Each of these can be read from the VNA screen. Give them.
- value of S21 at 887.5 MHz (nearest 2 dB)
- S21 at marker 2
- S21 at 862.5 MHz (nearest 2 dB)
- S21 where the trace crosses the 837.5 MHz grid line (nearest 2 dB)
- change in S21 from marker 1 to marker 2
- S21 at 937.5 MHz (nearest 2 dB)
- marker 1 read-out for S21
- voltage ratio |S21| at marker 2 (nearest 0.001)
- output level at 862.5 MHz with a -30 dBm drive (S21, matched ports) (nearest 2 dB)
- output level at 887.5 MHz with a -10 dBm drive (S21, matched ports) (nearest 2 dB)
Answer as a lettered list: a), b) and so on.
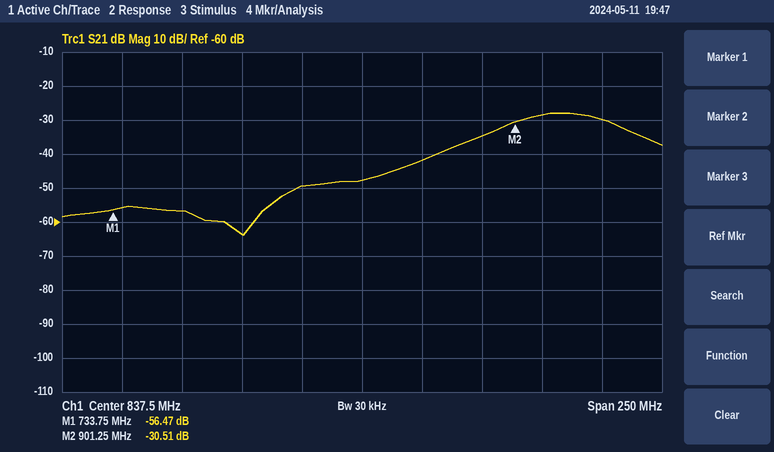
a) -34 dB
b) -30.51 dB
c) -42 dB
d) -48 dB
e) 25.96 dB
f) -30 dB
g) -56.47 dB
h) 0.030
i) -72 dBm
j) -44 dBm
